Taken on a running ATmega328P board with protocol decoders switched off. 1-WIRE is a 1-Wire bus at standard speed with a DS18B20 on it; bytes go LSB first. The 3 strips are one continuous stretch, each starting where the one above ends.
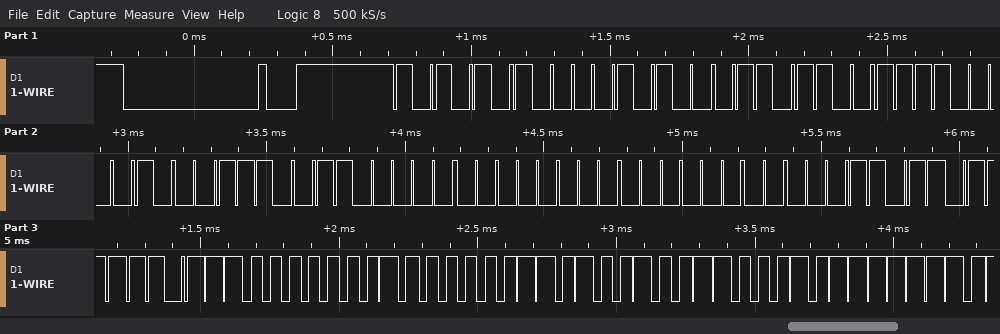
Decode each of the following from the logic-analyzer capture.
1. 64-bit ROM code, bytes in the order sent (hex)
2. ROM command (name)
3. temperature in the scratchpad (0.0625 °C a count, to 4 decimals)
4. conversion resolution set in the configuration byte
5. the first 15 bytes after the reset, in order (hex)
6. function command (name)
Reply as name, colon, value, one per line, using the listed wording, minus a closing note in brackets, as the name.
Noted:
64-bit ROM code, bytes in the order sent: 28 36 0F 71 06 00 00 D8
ROM command: Match ROM
temperature in the scratchpad: 32.1875 °C
conversion resolution set in the configuration byte: 12 bits
the first 15 bytes after the reset, in order: 55 28 36 0F 71 06 00 00 D8 BE 03 02 4B 46 7F
function command: Read Scratchpad
